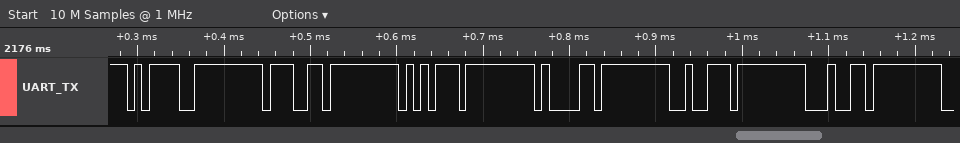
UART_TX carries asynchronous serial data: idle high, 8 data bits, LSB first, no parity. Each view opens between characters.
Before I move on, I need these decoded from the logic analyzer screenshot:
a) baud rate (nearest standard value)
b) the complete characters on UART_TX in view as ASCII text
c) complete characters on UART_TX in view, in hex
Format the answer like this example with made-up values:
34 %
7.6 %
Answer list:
115200 baud
"=guard"
3D, 67, 75, 61, 72, 64
